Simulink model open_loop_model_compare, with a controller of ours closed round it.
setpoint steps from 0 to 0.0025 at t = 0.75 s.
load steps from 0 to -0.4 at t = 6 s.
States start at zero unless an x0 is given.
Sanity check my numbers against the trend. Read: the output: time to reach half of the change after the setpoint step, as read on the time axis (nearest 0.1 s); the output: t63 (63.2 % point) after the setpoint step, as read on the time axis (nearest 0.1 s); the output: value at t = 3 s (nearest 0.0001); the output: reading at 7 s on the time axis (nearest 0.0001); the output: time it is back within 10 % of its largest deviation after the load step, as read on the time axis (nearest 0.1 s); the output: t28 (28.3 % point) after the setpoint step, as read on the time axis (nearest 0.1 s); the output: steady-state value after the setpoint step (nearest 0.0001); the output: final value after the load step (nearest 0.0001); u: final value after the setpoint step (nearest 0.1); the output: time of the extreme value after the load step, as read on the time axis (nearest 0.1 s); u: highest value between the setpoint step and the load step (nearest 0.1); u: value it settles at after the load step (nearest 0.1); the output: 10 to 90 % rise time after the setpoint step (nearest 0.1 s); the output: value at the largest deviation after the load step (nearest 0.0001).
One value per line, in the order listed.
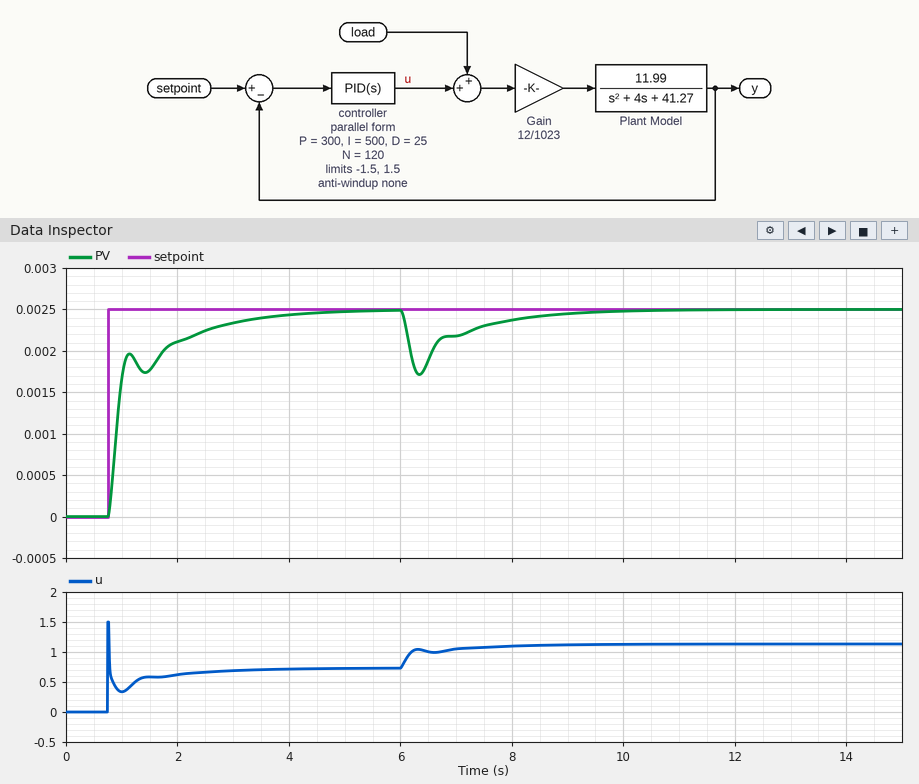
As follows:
0.9 s
1.0 s
0.0023
0.0022
8.6 s
0.9 s
0.0025
0.0025
0.7
6.3 s
1.5
1.1
1.7 s
0.0017
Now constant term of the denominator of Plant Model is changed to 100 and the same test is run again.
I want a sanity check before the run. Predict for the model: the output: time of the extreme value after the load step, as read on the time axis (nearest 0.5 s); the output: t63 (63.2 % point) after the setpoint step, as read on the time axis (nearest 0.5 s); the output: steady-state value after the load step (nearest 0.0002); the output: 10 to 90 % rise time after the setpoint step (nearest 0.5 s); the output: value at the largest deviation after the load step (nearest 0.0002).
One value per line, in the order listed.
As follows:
6.5 s
1.5 s
0.0016
2.0 s
0.0012
